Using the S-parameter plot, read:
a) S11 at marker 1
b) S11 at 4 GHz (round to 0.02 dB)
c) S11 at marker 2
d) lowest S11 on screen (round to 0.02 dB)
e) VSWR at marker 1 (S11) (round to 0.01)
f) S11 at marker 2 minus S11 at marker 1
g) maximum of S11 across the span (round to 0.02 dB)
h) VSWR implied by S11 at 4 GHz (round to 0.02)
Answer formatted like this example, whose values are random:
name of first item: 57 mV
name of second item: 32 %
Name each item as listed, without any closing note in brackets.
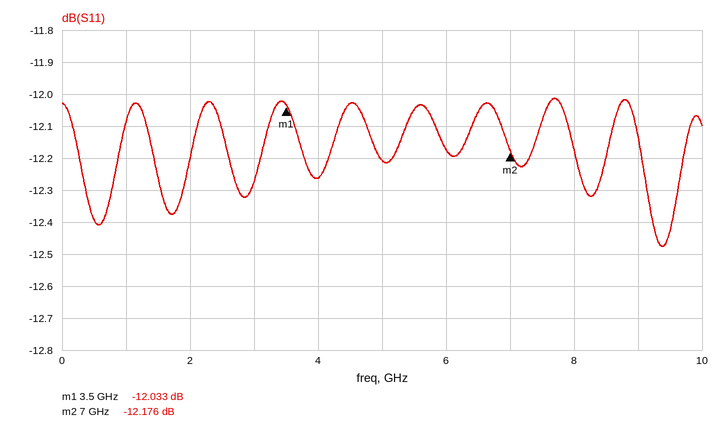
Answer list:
S11 at marker 1: -12.033 dB
S11 at 4 GHz: -12.26 dB
S11 at marker 2: -12.176 dB
lowest S11 on screen: -12.48 dB
VSWR at marker 1 (S11): 1.67
S11 at marker 2 minus S11 at marker 1: -0.143 dB
maximum of S11 across the span: -12.02 dB
VSWR implied by S11 at 4 GHz: 1.64
